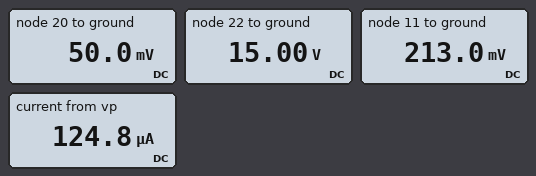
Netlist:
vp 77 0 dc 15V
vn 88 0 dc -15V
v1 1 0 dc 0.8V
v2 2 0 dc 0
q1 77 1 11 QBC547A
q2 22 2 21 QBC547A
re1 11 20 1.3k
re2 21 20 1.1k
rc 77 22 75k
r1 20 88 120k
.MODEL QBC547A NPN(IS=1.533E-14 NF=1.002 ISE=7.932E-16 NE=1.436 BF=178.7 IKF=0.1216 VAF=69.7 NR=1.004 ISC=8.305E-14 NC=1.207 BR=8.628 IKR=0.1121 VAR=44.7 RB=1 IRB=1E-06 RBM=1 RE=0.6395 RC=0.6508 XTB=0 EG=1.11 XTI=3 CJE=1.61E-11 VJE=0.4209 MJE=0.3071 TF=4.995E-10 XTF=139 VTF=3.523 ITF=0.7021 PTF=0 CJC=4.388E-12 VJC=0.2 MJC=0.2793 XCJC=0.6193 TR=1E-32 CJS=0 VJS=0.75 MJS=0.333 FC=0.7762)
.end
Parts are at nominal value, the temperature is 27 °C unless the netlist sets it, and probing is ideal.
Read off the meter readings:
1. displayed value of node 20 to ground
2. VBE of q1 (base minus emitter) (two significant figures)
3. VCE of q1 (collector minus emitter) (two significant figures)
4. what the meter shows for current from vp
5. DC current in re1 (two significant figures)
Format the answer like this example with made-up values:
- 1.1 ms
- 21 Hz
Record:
- 50.0 mV
- 590 mV
- 15 V
- 124.8 µA
- 130 µA
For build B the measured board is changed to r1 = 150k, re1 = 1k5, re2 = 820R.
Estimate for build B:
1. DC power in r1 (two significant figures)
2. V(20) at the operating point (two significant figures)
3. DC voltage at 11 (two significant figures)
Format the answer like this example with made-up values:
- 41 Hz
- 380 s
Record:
- 1.5 mW
- 68 mV
- 220 mV
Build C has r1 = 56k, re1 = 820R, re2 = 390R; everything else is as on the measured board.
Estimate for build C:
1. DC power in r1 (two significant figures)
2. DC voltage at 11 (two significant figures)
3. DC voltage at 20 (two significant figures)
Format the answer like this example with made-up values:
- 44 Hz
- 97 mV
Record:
- 4.0 mW
- 190 mV
- -26 mV
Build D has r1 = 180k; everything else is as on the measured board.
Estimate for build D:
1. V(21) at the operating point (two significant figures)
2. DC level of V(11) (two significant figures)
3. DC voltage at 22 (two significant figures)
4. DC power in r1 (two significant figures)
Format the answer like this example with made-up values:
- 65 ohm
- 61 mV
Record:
- 110 mV
- 220 mV
- 15 V
- 1.3 mW
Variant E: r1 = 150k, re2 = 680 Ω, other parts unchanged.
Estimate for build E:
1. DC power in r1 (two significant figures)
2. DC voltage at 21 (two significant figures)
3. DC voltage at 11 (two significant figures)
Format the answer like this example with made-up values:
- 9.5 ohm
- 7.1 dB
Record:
- 1.5 mW
- 88 mV
- 220 mV
